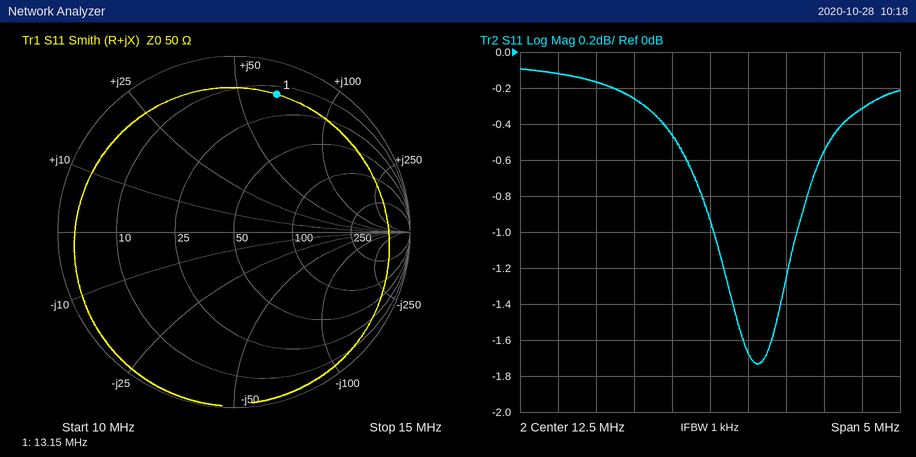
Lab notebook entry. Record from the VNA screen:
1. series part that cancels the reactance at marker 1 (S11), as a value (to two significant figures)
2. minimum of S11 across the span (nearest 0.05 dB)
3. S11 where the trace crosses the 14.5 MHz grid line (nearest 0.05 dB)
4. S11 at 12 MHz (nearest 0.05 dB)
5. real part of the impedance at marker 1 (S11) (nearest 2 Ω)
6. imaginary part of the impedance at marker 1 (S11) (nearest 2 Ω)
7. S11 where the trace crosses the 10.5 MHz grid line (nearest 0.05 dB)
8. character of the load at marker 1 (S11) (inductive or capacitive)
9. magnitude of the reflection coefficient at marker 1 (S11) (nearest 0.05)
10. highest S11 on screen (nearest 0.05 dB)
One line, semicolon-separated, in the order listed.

180 pF; -1.75 dB; -0.30 dB; -0.45 dB; 14 Ω; +66 Ω; -0.10 dB; inductive; 0.80; -0.10 dB
